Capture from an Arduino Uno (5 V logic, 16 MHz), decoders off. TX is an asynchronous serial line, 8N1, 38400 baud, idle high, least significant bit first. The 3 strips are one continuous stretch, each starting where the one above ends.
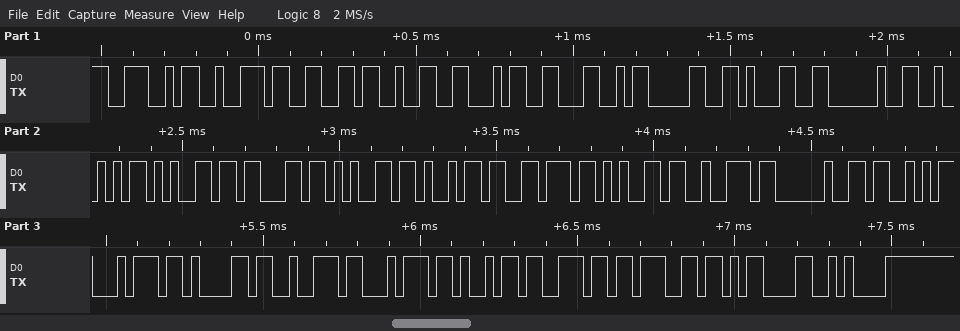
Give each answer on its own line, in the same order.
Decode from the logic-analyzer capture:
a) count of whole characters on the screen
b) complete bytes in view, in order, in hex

28
0x4E 0x72 0x66 0x32 0x34 0x4C 0x30 0x31 0x20 0x52 0x65 0x63 0x65 0x69 0x76 0x65 0x72 0x20 0x53 0x74 0x61 0x72 0x74 0x69 0x6E 0x67 0x0D 0x0A
